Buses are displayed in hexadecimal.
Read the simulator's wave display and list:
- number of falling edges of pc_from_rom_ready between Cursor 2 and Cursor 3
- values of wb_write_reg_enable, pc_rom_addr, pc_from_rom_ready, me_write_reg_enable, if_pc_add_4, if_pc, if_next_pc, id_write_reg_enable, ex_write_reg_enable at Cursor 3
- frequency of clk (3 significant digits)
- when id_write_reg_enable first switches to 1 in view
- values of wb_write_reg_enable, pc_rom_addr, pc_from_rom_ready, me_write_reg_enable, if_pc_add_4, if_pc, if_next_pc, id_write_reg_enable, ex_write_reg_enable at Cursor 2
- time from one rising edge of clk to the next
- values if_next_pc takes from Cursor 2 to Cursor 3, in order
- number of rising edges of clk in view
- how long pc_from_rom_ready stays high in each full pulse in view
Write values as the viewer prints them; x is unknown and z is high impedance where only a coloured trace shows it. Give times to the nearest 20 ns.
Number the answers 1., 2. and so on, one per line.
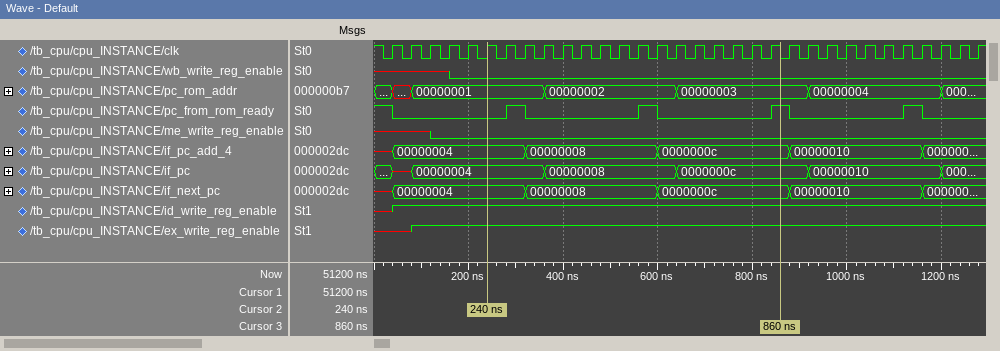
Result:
1. 2
2. wb_write_reg_enable=0, pc_rom_addr=00000003, pc_from_rom_ready=1, me_write_reg_enable=0, if_pc_add_4=0000000c, if_pc=0000000c, if_next_pc=0000000c, id_write_reg_enable=1, ex_write_reg_enable=1
3. 25.0 MHz
4. 40 ns
5. wb_write_reg_enable=0, pc_rom_addr=00000001, pc_from_rom_ready=0, me_write_reg_enable=0, if_pc_add_4=00000004, if_pc=00000004, if_next_pc=00000004, id_write_reg_enable=1, ex_write_reg_enable=1
6. 40 ns
7. 00000004, 00000008, 0000000c
8. 32
9. 40 ns, 40 ns, 40 ns, 40 ns
